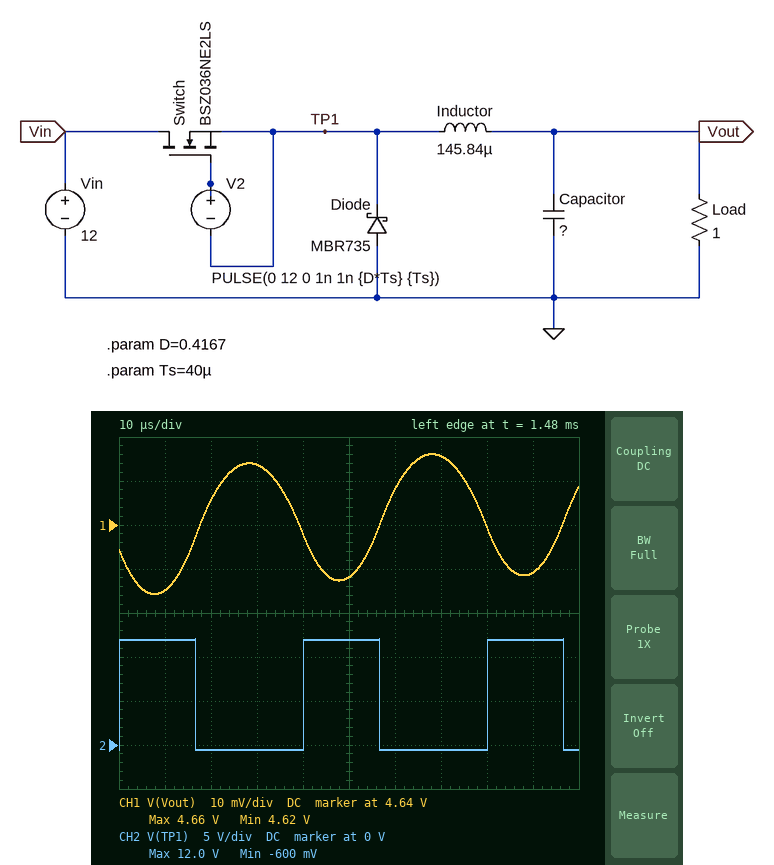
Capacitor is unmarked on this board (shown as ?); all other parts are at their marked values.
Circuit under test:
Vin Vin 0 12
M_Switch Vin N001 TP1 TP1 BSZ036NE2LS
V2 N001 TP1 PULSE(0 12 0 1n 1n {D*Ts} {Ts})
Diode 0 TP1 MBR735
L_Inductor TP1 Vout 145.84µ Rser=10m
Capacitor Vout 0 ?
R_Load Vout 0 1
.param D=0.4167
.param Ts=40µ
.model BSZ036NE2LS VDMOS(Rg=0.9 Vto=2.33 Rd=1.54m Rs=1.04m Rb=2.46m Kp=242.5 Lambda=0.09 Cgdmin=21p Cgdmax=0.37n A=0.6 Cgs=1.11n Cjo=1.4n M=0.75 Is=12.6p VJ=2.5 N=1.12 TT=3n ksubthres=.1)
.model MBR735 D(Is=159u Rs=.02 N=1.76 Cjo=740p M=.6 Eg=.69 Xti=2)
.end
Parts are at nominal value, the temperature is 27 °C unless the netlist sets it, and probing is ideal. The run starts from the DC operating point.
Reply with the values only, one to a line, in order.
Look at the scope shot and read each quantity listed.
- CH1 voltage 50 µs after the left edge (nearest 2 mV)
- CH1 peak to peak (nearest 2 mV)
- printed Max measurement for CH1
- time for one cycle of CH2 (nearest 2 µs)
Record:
4.628 V
32 mV
4.66 V
40 µs
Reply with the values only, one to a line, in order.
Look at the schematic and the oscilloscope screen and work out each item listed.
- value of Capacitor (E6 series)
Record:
150 µF
